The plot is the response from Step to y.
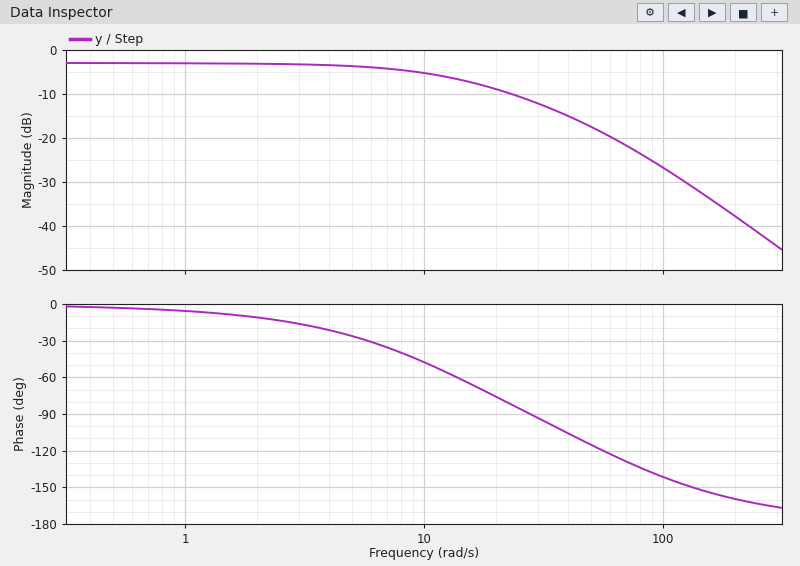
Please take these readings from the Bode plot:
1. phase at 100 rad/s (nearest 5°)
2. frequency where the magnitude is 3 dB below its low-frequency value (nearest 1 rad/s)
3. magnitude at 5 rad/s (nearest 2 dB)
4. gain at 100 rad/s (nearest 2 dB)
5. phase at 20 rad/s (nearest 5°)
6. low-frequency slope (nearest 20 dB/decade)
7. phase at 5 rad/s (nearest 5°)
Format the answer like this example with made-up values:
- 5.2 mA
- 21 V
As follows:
- -140°
- 12 rad/s
- -4 dB
- -26 dB
- -75°
- 0 dB/decade
- -25°
